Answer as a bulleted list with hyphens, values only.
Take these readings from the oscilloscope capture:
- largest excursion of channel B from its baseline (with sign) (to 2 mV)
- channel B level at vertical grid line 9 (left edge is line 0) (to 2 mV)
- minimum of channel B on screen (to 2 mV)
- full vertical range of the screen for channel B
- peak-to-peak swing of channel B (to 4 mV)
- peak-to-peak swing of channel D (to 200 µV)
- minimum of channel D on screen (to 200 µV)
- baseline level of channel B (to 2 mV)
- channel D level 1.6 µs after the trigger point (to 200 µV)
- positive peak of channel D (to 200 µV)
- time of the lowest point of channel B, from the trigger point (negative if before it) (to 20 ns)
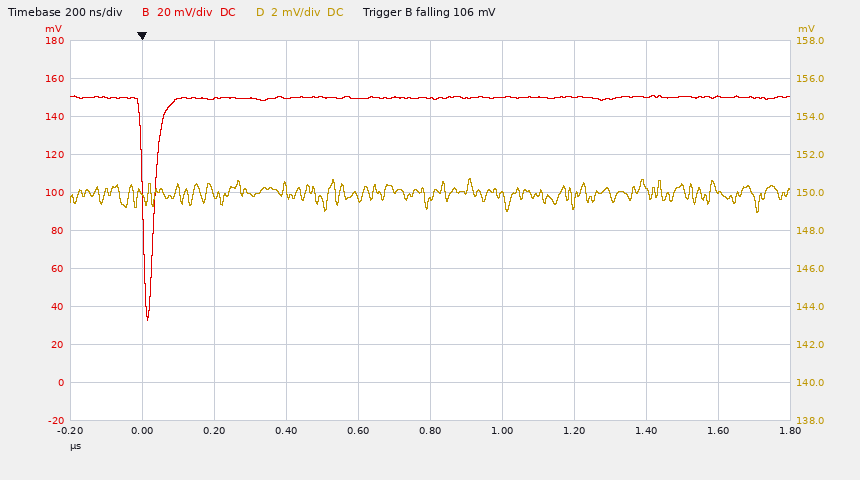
- -118 mV
- 150 mV
- 32 mV
- 200 mV
- 120 mV
- 1.8 mV
- 149.0 mV
- 150 mV
- 150.2 mV
- 150.8 mV
- +20 ns
